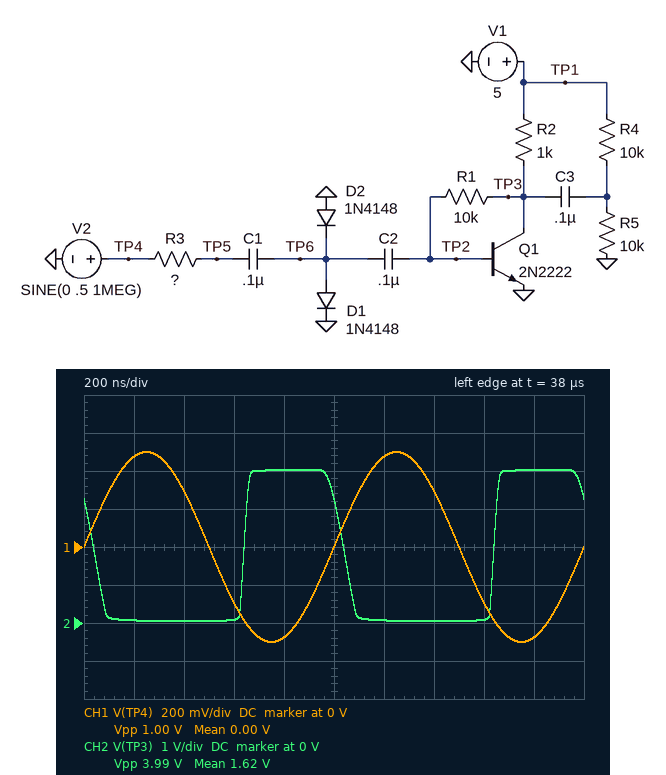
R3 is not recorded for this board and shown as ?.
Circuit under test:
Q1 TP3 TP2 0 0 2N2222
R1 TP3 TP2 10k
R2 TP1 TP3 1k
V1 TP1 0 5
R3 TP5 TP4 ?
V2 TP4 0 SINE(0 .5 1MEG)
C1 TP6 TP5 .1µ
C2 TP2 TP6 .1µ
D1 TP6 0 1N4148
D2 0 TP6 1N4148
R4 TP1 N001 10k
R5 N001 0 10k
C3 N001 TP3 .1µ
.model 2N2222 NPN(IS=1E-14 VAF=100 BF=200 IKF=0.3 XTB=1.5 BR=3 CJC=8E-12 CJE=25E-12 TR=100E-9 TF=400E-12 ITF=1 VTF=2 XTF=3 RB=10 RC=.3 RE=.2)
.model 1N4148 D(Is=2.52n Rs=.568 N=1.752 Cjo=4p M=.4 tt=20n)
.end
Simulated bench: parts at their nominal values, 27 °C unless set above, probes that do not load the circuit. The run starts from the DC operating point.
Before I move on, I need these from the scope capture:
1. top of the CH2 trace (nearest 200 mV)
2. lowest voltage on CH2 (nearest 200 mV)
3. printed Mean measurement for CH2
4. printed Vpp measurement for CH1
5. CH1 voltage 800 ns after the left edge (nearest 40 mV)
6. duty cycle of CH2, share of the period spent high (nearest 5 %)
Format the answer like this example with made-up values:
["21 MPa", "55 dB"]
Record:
["4.0 V", "0 V", "1.62 V", "1.00 V", "-480 mV", "40 %"]
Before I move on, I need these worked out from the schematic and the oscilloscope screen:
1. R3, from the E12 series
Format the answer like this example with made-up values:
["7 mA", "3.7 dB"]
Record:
["470 Ω"]
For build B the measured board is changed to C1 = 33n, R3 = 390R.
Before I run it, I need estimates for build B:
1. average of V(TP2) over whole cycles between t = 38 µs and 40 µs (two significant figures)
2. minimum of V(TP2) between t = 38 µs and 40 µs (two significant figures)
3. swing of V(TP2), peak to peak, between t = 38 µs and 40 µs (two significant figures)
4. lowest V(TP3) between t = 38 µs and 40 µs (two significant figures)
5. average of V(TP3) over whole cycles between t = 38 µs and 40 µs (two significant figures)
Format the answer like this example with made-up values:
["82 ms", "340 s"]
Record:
["580 mV", "250 mV", "470 mV", "47 mV", "1.8 V"]
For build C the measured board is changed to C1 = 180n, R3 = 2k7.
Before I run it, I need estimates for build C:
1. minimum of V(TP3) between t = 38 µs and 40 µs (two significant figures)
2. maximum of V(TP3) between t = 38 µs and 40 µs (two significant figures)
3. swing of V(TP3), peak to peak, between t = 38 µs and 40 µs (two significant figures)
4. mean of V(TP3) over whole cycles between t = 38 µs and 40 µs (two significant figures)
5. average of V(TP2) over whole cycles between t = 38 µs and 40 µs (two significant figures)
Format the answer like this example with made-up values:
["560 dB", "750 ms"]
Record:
["100 mV", "2.4 V", "2.3 V", "990 mV", "690 mV"]
